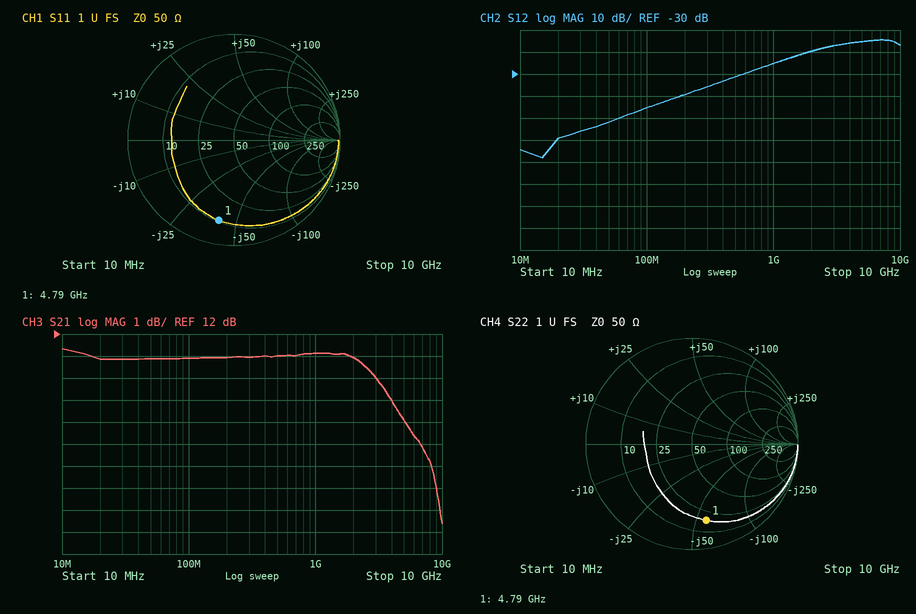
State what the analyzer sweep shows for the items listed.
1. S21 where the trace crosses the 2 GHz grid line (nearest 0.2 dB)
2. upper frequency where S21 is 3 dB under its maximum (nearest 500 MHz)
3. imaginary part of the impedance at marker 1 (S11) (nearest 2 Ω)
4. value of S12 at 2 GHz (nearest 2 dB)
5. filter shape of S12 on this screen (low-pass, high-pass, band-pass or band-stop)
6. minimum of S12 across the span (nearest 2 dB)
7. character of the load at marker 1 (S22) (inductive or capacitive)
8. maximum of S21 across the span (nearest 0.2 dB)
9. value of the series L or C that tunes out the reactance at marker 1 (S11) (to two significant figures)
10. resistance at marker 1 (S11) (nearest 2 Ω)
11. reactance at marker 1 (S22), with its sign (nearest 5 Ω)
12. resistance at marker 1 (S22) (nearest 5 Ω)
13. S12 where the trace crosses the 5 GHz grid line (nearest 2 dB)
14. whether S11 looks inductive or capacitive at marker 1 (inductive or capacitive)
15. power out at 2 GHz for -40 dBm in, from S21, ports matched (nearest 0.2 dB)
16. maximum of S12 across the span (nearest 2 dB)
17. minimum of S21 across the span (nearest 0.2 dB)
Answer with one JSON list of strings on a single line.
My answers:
["11.0 dB", "4.5 GHz", "-40 Ω", "-20 dB", "high-pass", "-68 dB", "capacitive", "11.4 dB", "1.3 nH", "10 Ω", "-55 Ω", "20 Ω", "-16 dB", "capacitive", "-29.0 dBm", "-14 dB", "3.4 dB"]
